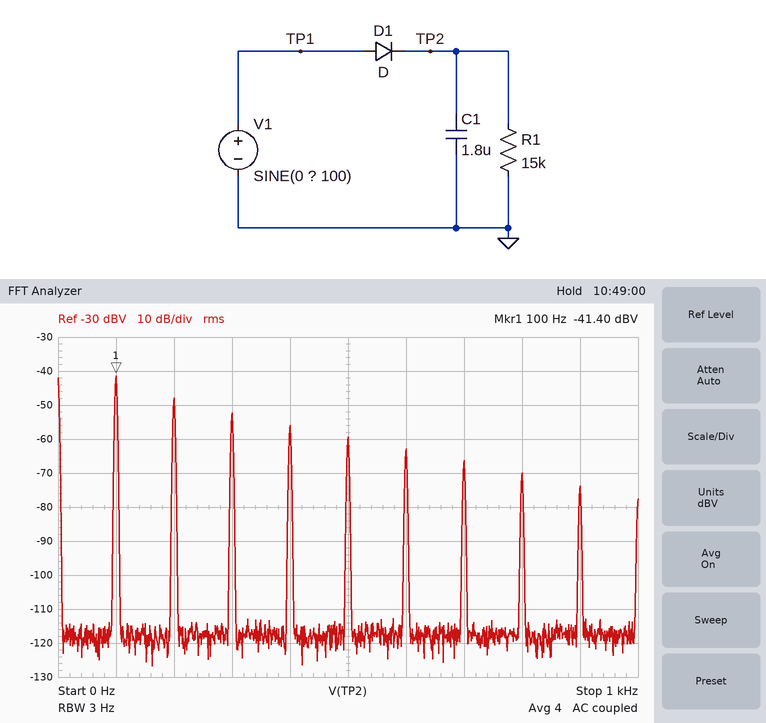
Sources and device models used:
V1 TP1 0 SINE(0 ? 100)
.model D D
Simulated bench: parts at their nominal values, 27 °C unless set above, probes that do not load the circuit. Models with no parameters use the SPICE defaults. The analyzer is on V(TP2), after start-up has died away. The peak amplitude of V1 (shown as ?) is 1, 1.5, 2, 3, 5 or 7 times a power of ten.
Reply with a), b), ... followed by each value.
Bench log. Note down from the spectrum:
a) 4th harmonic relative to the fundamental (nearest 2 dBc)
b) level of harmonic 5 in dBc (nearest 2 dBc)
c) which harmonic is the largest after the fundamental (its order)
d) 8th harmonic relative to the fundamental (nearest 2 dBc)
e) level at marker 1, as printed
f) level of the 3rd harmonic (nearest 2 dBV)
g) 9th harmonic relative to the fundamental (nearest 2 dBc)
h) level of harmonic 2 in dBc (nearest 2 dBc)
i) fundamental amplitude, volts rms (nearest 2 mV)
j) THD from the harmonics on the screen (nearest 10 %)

a) -14 dBc
b) -18 dBc
c) 2
d) -28 dBc
e) -41.40 dBV
f) -52 dBV
g) -32 dBc
h) -6 dBc
i) 8 mV
j) 60 %
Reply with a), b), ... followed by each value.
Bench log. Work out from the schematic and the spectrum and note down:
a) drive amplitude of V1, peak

a) 700 mV
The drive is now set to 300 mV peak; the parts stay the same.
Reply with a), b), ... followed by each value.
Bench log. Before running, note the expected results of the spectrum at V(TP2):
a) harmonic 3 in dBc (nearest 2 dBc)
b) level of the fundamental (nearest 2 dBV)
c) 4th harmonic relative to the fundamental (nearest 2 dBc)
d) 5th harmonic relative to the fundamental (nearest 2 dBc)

a) -12 dBc
b) -136 dBV
c) -18 dBc
d) -24 dBc
